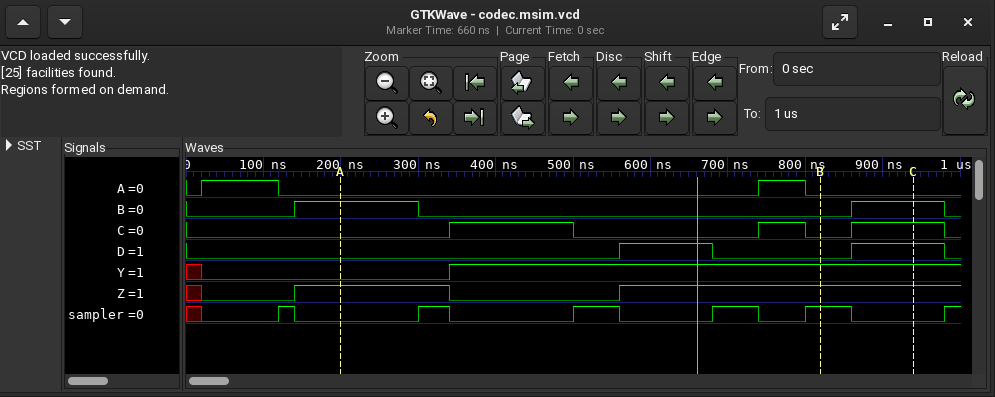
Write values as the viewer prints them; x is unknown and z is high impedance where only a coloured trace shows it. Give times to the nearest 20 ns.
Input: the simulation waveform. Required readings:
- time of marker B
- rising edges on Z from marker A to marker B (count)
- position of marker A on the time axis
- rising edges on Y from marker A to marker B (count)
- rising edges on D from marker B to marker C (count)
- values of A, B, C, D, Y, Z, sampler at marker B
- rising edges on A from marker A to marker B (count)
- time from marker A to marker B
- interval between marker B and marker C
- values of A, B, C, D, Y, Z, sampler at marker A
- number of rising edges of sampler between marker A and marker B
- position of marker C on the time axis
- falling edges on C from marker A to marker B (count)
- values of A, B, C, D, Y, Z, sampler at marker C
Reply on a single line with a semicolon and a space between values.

820 ns; 1; 200 ns; 1; 1; A=0, B=0, C=0, D=0, Y=1, Z=1, sampler=1; 1; 620 ns; 120 ns; A=0, B=1, C=0, D=0, Y=0, Z=1, sampler=0; 4; 940 ns; 2; A=0, B=1, C=1, D=1, Y=1, Z=1, sampler=0
